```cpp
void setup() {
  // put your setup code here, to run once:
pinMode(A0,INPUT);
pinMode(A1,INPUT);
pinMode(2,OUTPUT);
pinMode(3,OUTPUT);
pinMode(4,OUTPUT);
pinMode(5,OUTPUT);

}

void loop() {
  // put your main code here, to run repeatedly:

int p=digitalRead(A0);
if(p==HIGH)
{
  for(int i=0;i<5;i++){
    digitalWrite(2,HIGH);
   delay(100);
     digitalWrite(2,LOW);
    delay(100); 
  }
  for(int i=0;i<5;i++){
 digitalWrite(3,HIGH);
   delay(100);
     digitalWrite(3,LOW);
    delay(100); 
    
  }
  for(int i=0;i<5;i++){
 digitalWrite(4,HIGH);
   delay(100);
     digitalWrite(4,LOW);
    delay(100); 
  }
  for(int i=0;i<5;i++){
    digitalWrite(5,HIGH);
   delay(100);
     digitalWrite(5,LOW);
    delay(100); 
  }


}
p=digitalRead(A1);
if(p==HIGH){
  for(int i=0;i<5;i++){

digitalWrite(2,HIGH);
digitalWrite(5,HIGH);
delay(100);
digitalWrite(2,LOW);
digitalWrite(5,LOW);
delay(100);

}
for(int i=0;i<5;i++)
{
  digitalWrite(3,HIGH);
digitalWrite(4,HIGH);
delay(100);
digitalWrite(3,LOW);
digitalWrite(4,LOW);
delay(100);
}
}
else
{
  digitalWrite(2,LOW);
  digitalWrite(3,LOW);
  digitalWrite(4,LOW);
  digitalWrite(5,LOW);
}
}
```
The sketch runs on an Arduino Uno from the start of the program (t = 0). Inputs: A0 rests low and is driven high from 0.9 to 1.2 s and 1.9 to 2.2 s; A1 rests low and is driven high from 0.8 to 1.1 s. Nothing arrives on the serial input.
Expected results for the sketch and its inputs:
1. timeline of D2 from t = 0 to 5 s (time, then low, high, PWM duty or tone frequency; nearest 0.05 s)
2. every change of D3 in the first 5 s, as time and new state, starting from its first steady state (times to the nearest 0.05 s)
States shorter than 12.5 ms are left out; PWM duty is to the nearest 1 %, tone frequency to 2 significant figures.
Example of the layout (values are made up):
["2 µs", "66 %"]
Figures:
["0 s low; 0.8 s high; 0.9 s low; 1 s high; 1.1 s low; 1.2 s high; 1.3 s low; 1.4 s high; 1.5 s low; 1.6 s high; 1.7 s low", "0 s low; 1.8 s high; 1.9 s low; 2 s high; 2.1 s low; 2.2 s high; 2.3 s low; 2.4 s high; 2.5 s low; 2.6 s high; 2.7 s low"]
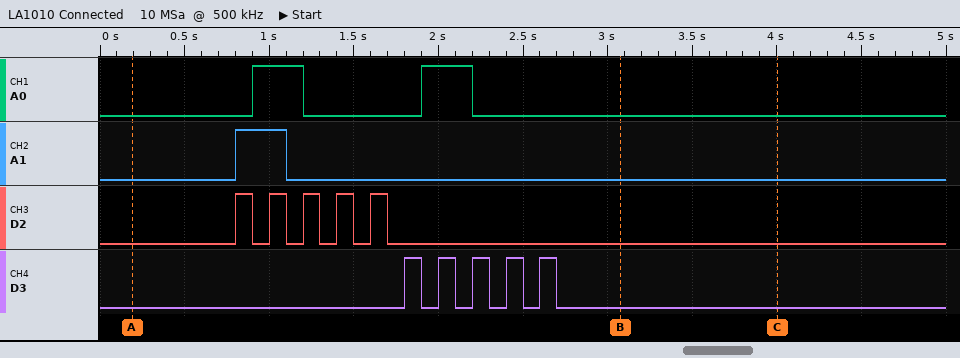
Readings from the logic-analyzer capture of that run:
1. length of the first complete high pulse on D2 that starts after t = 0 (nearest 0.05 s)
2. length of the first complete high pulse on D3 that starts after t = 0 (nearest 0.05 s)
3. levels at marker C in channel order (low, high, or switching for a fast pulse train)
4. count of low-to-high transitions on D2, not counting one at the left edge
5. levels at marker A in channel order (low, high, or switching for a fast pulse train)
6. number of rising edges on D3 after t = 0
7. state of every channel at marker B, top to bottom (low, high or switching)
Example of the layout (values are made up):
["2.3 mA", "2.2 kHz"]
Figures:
["0.10 s", "0.10 s", "A0 low, A1 low, D2 low, D3 low", "5", "A0 low, A1 low, D2 low, D3 low", "5", "A0 low, A1 low, D2 low, D3 low"]
